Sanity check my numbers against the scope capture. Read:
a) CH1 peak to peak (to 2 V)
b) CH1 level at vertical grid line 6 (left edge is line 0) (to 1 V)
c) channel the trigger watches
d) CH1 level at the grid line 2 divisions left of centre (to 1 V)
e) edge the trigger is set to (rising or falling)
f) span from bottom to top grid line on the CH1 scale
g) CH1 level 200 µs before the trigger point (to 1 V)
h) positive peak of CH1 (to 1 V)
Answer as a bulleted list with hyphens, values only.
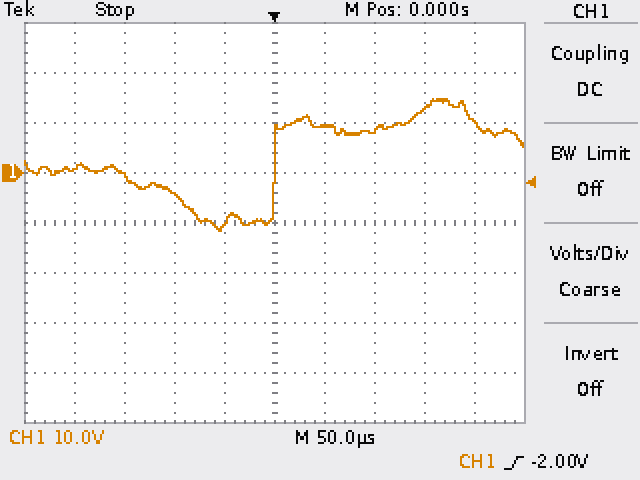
- 26 V
- 9 V
- CH1
- -4 V
- rising
- 80 V
- 1 V
- 15 V
